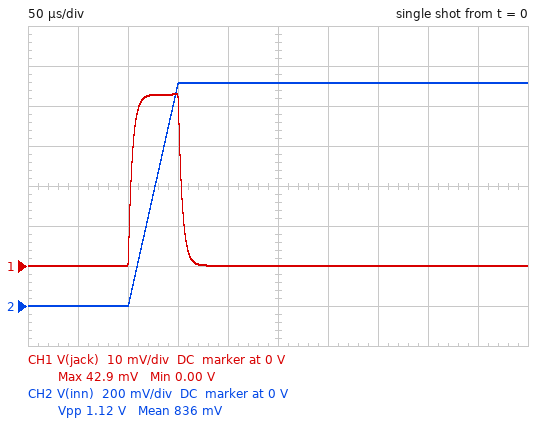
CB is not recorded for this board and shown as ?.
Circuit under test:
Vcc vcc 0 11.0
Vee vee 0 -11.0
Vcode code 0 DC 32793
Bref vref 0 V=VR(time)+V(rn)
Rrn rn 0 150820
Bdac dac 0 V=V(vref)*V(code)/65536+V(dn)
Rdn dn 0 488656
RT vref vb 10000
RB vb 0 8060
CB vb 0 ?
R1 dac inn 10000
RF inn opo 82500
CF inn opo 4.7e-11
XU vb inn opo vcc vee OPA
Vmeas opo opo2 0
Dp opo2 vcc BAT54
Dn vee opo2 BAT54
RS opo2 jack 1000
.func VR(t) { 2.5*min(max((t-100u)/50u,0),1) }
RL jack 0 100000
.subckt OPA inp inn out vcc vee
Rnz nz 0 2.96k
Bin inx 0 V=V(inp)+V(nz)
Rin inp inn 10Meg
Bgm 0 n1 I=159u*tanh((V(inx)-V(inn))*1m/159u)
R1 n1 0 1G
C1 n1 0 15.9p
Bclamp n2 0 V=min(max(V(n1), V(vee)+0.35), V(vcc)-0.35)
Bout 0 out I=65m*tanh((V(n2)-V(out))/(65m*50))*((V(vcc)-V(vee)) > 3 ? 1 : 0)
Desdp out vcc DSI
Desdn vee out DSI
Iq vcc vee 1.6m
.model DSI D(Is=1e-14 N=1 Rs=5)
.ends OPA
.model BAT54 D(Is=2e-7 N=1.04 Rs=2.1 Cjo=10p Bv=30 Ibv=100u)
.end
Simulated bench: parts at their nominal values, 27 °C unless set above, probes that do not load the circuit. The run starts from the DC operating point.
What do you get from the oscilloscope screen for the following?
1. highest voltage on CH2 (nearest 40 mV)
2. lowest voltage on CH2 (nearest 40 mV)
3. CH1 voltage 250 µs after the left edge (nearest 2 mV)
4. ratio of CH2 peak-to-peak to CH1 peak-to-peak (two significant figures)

1.12 V
0 V
0 V
26
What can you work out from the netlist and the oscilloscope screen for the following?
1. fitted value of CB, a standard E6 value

47 pF
